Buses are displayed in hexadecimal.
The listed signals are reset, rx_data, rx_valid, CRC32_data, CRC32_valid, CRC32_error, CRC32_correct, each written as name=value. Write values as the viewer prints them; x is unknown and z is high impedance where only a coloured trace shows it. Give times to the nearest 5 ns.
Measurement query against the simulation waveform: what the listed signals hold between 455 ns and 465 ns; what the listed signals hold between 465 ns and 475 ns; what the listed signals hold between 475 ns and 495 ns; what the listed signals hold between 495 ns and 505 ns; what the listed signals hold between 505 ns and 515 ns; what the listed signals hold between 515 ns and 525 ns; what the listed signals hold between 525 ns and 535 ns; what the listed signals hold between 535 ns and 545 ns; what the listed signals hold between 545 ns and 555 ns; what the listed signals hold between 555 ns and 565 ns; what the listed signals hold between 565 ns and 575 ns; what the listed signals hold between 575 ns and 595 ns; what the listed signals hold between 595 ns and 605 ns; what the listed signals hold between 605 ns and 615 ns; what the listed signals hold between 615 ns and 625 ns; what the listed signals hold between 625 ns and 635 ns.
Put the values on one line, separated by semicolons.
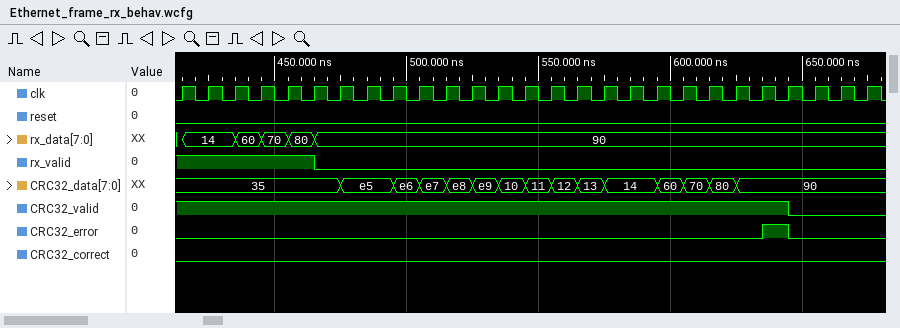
reset=0, rx_data=80, rx_valid=1, CRC32_data=35, CRC32_valid=1, CRC32_error=0, CRC32_correct=0; reset=0, rx_data=90, rx_valid=0, CRC32_data=35, CRC32_valid=1, CRC32_error=0, CRC32_correct=0; reset=0, rx_data=90, rx_valid=0, CRC32_data=e5, CRC32_valid=1, CRC32_error=0, CRC32_correct=0; reset=0, rx_data=90, rx_valid=0, CRC32_data=e6, CRC32_valid=1, CRC32_error=0, CRC32_correct=0; reset=0, rx_data=90, rx_valid=0, CRC32_data=e7, CRC32_valid=1, CRC32_error=0, CRC32_correct=0; reset=0, rx_data=90, rx_valid=0, CRC32_data=e8, CRC32_valid=1, CRC32_error=0, CRC32_correct=0; reset=0, rx_data=90, rx_valid=0, CRC32_data=e9, CRC32_valid=1, CRC32_error=0, CRC32_correct=0; reset=0, rx_data=90, rx_valid=0, CRC32_data=10, CRC32_valid=1, CRC32_error=0, CRC32_correct=0; reset=0, rx_data=90, rx_valid=0, CRC32_data=11, CRC32_valid=1, CRC32_error=0, CRC32_correct=0; reset=0, rx_data=90, rx_valid=0, CRC32_data=12, CRC32_valid=1, CRC32_error=0, CRC32_correct=0; reset=0, rx_data=90, rx_valid=0, CRC32_data=13, CRC32_valid=1, CRC32_error=0, CRC32_correct=0; reset=0, rx_data=90, rx_valid=0, CRC32_data=14, CRC32_valid=1, CRC32_error=0, CRC32_correct=0; reset=0, rx_data=90, rx_valid=0, CRC32_data=60, CRC32_valid=1, CRC32_error=0, CRC32_correct=0; reset=0, rx_data=90, rx_valid=0, CRC32_data=70, CRC32_valid=1, CRC32_error=0, CRC32_correct=0; reset=0, rx_data=90, rx_valid=0, CRC32_data=80, CRC32_valid=1, CRC32_error=0, CRC32_correct=0; reset=0, rx_data=90, rx_valid=0, CRC32_data=90, CRC32_valid=1, CRC32_error=0, CRC32_correct=0
